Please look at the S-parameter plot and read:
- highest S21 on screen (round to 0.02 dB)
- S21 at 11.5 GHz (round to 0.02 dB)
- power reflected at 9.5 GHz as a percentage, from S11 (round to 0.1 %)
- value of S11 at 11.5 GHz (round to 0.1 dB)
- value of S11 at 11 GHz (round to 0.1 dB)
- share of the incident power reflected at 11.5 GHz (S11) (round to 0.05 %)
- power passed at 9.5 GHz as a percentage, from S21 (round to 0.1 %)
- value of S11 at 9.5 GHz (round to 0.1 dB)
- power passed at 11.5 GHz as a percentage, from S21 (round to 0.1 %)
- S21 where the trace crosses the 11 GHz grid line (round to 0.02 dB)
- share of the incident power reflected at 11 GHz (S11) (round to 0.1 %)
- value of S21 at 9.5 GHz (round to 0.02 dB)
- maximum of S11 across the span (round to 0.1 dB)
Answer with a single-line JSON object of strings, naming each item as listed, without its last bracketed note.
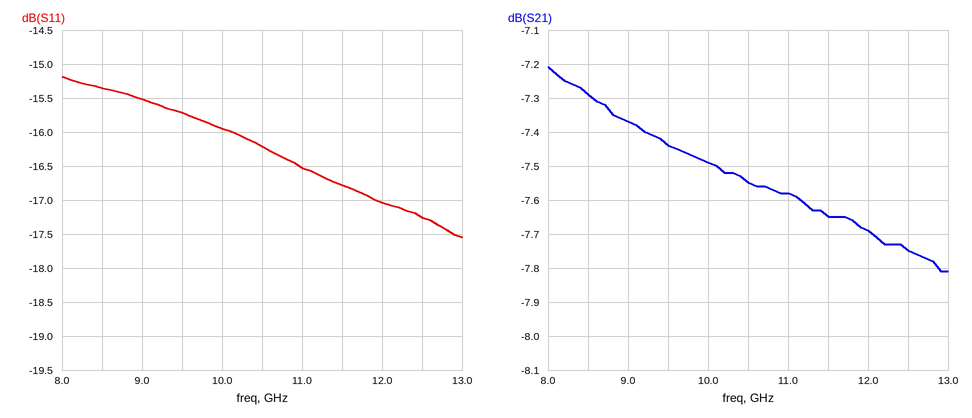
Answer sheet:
{"highest S21 on screen": "-7.20 dB", "S21 at 11.5 GHz": "-7.64 dB", "power reflected at 9.5 GHz as a percentage, from S11": "2.7 %", "value of S11 at 11.5 GHz": "-16.8 dB", "value of S11 at 11 GHz": "-16.5 dB", "share of the incident power reflected at 11.5 GHz (S11)": "2.10 %", "power passed at 9.5 GHz as a percentage, from S21": "18.0 %", "value of S11 at 9.5 GHz": "-15.7 dB", "power passed at 11.5 GHz as a percentage, from S21": "17.2 %", "S21 where the trace crosses the 11 GHz grid line": "-7.58 dB", "share of the incident power reflected at 11 GHz (S11)": "2.2 %", "value of S21 at 9.5 GHz": "-7.44 dB", "maximum of S11 across the span": "-15.2 dB"}
